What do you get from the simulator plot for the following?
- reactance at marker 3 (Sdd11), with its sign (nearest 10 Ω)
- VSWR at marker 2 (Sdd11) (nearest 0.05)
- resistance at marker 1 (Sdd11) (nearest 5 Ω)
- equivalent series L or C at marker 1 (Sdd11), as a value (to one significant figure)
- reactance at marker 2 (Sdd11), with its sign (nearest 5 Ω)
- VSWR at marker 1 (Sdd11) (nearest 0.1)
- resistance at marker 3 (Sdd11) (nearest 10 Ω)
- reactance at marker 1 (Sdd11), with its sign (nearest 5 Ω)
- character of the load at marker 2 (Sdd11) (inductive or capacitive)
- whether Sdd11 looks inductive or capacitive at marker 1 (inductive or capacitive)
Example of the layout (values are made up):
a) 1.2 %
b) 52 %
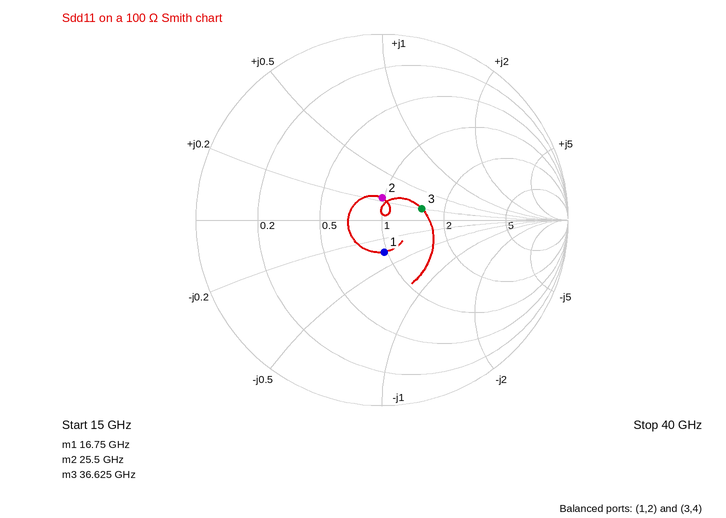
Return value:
a) +20 Ω
b) 1.25
c) 95 Ω
d) 300 fF
e) +25 Ω
f) 1.4
g) 150 Ω
h) -35 Ω
i) inductive
j) capacitive
